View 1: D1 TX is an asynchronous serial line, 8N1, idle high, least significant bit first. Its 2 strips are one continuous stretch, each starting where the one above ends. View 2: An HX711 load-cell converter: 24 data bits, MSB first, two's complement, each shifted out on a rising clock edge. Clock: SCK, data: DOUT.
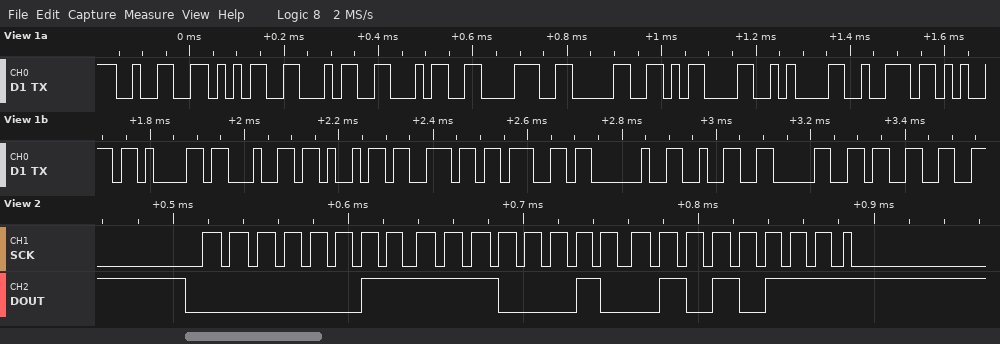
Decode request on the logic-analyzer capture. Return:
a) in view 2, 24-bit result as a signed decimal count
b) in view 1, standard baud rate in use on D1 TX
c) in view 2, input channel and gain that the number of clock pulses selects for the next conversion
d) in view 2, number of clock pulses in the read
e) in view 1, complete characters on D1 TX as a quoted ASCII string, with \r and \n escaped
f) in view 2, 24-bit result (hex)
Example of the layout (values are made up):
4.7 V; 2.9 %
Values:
254551; 57600 baud; channel A, gain 128; 25; "254480\r\nreading 203"; 0x03E257
